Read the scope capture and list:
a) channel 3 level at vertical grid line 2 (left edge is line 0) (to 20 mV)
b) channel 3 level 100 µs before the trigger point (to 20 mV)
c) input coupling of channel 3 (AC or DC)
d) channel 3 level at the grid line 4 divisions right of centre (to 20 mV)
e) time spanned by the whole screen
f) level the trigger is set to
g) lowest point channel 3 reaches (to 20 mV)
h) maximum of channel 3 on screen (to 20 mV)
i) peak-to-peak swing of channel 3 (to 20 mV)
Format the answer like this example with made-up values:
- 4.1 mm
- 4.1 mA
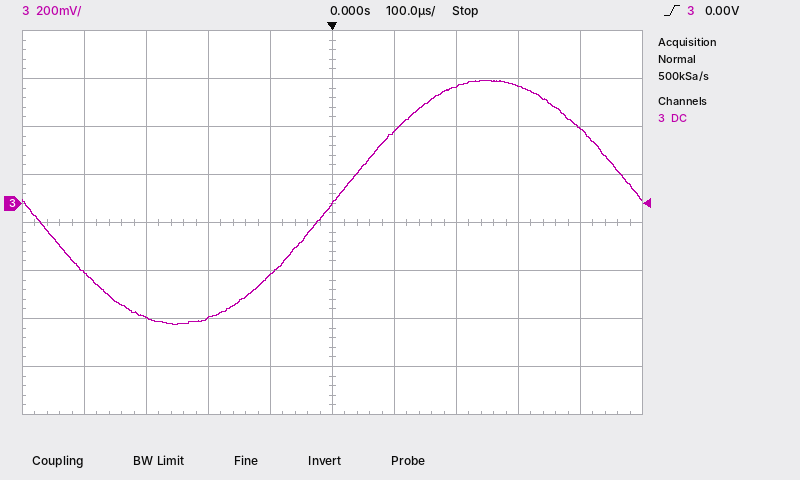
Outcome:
- -480 mV
- -300 mV
- DC
- 320 mV
- 1 ms
- 0.00 V
- -500 mV
- 520 mV
- 1.02 V
